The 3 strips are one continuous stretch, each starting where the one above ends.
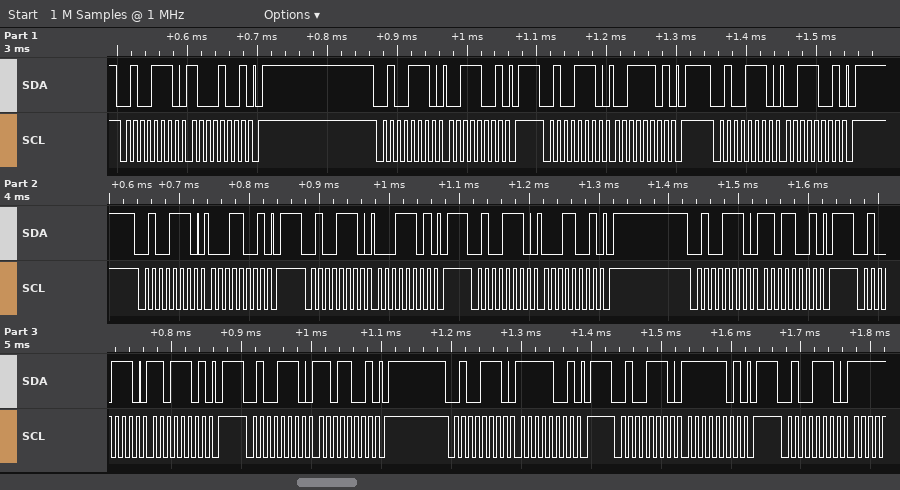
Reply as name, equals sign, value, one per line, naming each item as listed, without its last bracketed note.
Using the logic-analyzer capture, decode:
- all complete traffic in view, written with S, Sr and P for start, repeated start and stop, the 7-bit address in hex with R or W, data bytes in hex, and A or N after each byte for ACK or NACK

all complete traffic in view, written with S, Sr and P for start, repeated start and stop, the 7-bit address in hex with R or W, data bytes in hex, and A or N after each byte for ACK or NACK = S 27W A 89 A P S 27W A 39 A P S 27W A 3D A P S 27W A 39 A P S 27W A 19 A P S 27W A 1D A P S 27W A 19 A P S 27W A D9 A P S 27W A DD A P S 27W A D9 A P S 27W A F9 A P S 27W A FD A P S 27W A
